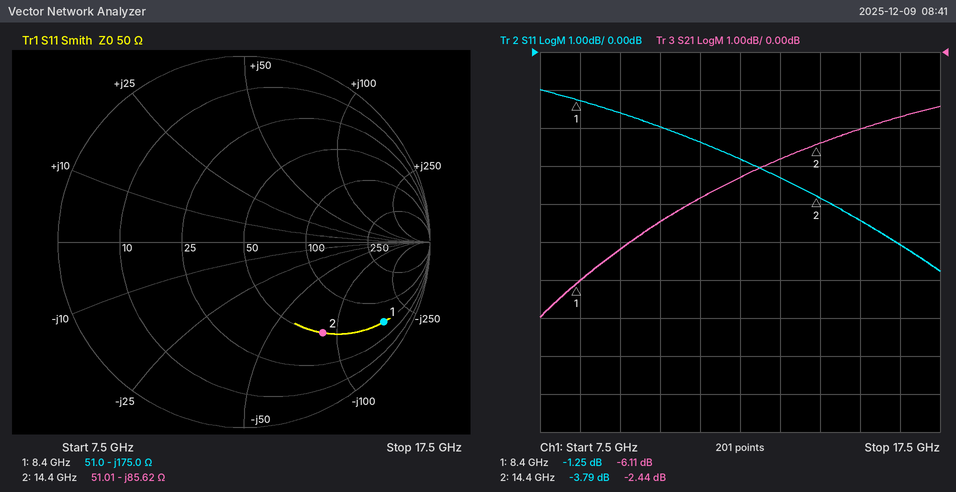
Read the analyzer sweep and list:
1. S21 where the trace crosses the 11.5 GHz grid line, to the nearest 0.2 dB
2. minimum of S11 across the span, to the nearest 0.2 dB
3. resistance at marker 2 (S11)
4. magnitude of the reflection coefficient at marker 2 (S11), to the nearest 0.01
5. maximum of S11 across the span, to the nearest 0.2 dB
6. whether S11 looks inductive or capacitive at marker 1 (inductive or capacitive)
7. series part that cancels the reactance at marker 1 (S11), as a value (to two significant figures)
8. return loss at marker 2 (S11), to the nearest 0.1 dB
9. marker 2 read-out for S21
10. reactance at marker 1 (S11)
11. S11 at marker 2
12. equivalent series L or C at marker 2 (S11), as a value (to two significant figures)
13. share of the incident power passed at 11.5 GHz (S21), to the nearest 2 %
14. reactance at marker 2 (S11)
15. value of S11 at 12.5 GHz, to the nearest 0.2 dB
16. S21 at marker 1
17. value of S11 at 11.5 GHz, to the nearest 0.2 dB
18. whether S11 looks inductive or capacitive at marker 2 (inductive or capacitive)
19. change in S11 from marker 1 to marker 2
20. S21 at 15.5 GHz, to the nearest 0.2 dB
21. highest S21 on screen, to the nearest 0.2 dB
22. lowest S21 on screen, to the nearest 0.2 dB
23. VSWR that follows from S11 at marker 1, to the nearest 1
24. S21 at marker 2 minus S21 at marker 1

-3.8 dB
-5.8 dB
51.01 Ω
0.65
-1.0 dB
capacitive
3.3 nH
3.8 dB
-2.44 dB
-175.0 Ω
-3.79 dB
130 fF
42 %
-85.62 Ω
-2.8 dB
-6.11 dB
-2.4 dB
capacitive
-2.54 dB
-2.0 dB
-1.4 dB
-7.0 dB
14
3.67 dB
